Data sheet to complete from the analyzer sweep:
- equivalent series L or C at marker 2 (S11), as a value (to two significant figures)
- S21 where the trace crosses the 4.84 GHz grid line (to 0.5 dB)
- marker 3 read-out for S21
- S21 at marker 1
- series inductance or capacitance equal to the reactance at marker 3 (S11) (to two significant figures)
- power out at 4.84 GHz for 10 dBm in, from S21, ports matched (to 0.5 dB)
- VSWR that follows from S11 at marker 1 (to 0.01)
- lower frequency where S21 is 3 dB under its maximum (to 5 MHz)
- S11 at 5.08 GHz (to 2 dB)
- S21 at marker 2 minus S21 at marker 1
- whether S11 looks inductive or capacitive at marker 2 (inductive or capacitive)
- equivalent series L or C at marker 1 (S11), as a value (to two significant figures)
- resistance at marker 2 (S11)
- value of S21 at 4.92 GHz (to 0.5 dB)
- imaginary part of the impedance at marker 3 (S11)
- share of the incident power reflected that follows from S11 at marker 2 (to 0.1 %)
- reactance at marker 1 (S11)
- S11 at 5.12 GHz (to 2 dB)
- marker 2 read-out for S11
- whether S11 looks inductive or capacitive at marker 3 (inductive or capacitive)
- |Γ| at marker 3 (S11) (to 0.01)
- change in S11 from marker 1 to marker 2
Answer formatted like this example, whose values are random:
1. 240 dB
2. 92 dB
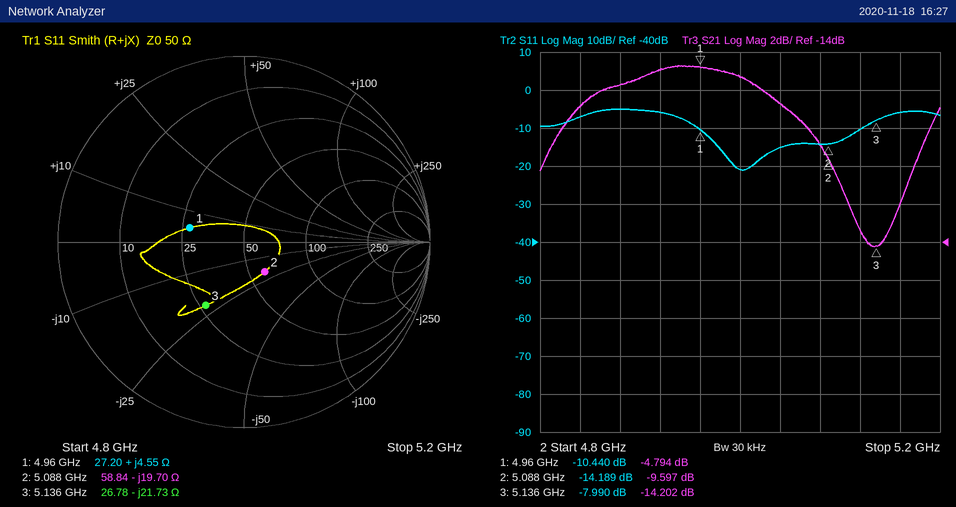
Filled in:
1. 1.6 pF
2. -7.0 dB
3. -14.202 dB
4. -4.794 dB
5. 1.4 pF
6. 3.0 dBm
7. 1.86
8. 4.825 GHz
9. -14 dB
10. -4.803 dB
11. capacitive
12. 150 pH
13. 58.84 Ω
14. -5.0 dB
15. -21.73 Ω
16. 3.8 %
17. +4.55 Ω
18. -10 dB
19. -14.189 dB
20. capacitive
21. 0.40
22. -3.749 dB
